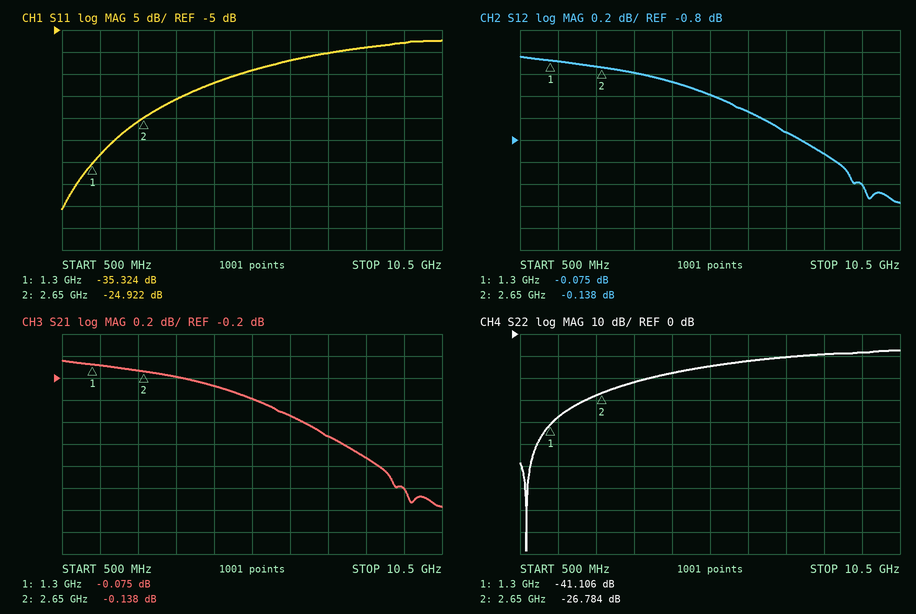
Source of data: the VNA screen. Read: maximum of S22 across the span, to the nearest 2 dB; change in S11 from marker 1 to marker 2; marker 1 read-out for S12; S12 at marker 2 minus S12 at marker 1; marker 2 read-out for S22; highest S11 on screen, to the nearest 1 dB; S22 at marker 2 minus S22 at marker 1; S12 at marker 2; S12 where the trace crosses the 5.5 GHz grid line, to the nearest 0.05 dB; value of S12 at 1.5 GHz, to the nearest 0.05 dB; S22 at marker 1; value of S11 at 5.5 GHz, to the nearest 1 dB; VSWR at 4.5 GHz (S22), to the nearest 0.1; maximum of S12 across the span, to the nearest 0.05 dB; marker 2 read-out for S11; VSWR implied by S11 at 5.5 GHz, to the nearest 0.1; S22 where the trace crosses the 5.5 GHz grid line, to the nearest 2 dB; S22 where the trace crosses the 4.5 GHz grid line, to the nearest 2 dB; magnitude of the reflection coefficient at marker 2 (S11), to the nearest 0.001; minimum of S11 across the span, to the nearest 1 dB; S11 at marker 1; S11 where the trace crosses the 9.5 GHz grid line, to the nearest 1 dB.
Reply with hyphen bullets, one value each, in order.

- -8 dB
- 10.402 dB
- -0.075 dB
- -0.063 dB
- -26.784 dB
- -7 dB
- 14.322 dB
- -0.138 dB
- -0.40 dB
- -0.10 dB
- -41.106 dB
- -14 dB
- 1.3
- -0.05 dB
- -24.922 dB
- 1.5
- -14 dB
- -18 dB
- 0.057
- -46 dB
- -35.324 dB
- -8 dB
